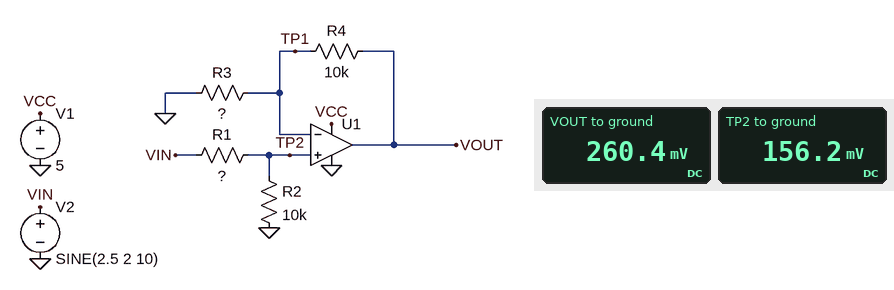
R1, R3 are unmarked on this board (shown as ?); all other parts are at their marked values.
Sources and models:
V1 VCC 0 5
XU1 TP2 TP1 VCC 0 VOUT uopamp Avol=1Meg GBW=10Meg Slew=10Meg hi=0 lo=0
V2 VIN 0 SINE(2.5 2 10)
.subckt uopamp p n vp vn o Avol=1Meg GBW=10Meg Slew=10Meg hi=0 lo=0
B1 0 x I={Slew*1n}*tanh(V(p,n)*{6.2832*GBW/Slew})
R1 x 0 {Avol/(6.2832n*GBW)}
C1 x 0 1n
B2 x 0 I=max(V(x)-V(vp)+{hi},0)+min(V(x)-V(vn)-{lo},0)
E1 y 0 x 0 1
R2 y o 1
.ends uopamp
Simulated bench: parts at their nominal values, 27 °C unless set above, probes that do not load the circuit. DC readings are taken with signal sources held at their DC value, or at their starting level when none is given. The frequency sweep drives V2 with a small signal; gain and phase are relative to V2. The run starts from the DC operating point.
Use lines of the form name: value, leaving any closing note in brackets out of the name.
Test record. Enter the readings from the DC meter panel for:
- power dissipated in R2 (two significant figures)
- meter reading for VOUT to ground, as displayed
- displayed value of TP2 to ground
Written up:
power dissipated in R2: 2.4 µW
meter reading for VOUT to ground, as displayed: 260.4 mV
displayed value of TP2 to ground: 156.2 mV
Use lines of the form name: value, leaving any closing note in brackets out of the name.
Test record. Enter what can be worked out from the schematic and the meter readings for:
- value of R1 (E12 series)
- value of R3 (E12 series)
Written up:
value of R1: 150 kΩ
value of R3: 15 kΩ
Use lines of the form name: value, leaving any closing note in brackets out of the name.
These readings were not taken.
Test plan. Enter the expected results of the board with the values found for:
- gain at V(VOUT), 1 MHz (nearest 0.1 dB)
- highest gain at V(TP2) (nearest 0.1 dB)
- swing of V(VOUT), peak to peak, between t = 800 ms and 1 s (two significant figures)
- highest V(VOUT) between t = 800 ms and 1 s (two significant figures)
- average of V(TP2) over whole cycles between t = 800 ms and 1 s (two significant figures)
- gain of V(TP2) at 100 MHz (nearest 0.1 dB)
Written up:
gain at V(VOUT), 1 MHz: -19.8 dB
highest gain at V(TP2): -24.1 dB
swing of V(VOUT), peak to peak, between t = 800 ms and 1 s: 420 mV
highest V(VOUT) between t = 800 ms and 1 s: 470 mV
average of V(TP2) over whole cycles between t = 800 ms and 1 s: 160 mV
gain of V(TP2) at 100 MHz: -24.1 dB
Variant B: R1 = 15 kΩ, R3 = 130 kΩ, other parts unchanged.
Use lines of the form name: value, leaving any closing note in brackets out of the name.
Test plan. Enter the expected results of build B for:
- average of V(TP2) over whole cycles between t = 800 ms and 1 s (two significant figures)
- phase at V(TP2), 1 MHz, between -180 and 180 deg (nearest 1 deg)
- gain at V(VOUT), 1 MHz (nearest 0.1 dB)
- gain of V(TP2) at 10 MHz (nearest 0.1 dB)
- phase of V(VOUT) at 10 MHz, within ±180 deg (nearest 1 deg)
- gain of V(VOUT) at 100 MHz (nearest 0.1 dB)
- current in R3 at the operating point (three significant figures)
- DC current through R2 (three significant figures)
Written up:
average of V(TP2) over whole cycles between t = 800 ms and 1 s: 1.0 V
phase at V(TP2), 1 MHz, between -180 and 180 deg: 0 deg
gain at V(VOUT), 1 MHz: -7.4 dB
gain of V(TP2) at 10 MHz: -8.0 dB
phase of V(VOUT) at 10 MHz, within ±180 deg: -47 deg
gain of V(VOUT) at 100 MHz: -28.0 dB
current in R3 at the operating point: 7.69 µA
DC current through R2: 100 µA
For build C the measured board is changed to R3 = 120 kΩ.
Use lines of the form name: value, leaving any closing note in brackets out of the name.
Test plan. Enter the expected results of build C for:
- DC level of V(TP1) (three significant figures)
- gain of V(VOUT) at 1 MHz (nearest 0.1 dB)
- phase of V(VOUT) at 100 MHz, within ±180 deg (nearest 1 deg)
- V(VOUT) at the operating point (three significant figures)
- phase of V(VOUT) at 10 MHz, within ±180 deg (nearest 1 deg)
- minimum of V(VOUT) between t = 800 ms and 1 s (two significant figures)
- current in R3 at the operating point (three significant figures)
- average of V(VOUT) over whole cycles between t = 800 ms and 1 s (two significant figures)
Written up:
DC level of V(TP1): 156 mV
gain of V(VOUT) at 1 MHz: -23.4 dB
phase of V(VOUT) at 100 MHz, within ±180 deg: -85 deg
V(VOUT) at the operating point: 169 mV
phase of V(VOUT) at 10 MHz, within ±180 deg: -47 deg
minimum of V(VOUT) between t = 800 ms and 1 s: 34 mV
current in R3 at the operating point: 1.30 µA
average of V(VOUT) over whole cycles between t = 800 ms and 1 s: 170 mV
